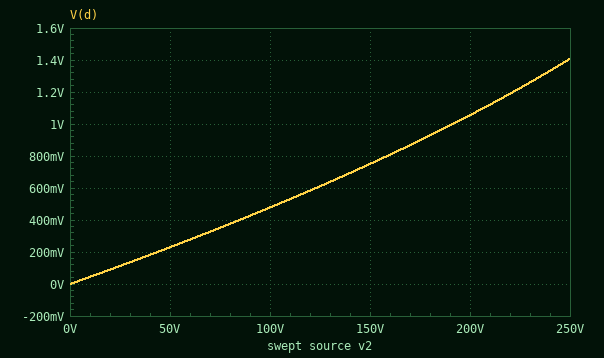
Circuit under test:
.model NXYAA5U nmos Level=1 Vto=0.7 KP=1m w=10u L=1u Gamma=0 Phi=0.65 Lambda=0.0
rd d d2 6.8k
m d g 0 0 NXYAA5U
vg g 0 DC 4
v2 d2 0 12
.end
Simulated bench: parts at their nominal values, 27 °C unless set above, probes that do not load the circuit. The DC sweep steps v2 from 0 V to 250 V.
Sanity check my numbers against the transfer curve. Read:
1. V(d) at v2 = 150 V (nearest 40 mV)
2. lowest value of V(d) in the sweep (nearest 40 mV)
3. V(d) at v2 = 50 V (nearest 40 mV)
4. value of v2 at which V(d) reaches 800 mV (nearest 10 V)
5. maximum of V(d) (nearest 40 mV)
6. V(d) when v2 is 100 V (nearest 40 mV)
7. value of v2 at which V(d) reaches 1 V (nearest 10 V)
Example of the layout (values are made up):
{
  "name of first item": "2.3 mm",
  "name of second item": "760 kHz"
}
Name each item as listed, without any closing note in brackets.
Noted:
{
  "V(d) at v2 = 150 V": "760 mV",
  "lowest value of V(d) in the sweep": "0 V",
  "V(d) at v2 = 50 V": "240 mV",
  "value of v2 at which V(d) reaches 800 mV": "160 V",
  "maximum of V(d)": "1.40 V",
  "V(d) when v2 is 100 V": "480 mV",
  "value of v2 at which V(d) reaches 1 V": "190 V"
}
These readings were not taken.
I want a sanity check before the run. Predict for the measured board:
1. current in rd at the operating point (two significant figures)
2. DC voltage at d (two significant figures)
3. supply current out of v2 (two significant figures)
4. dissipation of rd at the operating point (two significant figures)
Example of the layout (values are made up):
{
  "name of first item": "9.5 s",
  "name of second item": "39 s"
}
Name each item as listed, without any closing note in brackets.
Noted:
{
  "current in rd at the operating point": "1.8 mA",
  "DC voltage at d": "54 mV",
  "supply current out of v2": "1.8 mA",
  "dissipation of rd at the operating point": "21 mW"
}
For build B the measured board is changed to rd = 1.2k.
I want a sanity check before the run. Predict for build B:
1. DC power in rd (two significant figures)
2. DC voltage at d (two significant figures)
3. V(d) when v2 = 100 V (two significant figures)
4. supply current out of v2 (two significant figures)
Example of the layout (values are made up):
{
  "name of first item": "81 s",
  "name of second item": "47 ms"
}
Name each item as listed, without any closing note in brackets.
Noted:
{
  "DC power in rd": "110 mW",
  "DC voltage at d": "310 mV",
  "V(d) when v2 = 100 V": "35 V",
  "supply current out of v2": "9.7 mA"
}
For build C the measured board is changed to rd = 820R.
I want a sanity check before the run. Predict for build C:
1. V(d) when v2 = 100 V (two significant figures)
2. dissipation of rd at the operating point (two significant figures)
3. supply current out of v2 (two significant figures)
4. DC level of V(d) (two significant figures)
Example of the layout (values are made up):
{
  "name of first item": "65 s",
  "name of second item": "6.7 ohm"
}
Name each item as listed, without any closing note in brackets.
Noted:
{
  "V(d) when v2 = 100 V": "55 V",
  "dissipation of rd at the operating point": "160 mW",
  "supply current out of v2": "14 mA",
  "DC level of V(d)": "460 mV"
}
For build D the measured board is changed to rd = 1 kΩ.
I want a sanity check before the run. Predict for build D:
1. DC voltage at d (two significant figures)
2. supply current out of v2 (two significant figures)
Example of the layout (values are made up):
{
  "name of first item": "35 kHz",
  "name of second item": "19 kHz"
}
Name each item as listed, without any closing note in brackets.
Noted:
{
  "DC voltage at d": "370 mV",
  "supply current out of v2": "12 mA"
}
